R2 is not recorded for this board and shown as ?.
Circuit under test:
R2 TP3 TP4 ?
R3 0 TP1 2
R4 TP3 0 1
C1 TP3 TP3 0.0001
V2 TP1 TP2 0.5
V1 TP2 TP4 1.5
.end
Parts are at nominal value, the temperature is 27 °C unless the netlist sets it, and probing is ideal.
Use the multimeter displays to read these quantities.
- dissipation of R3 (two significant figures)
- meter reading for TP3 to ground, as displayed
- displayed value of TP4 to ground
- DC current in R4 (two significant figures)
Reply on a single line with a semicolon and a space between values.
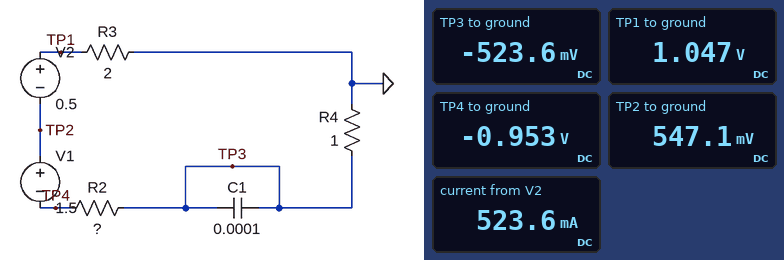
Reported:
550 mW; -523.6 mV; -0.953 V; 520 mA
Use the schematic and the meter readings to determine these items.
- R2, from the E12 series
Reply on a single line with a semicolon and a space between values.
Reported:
0.82 Ω
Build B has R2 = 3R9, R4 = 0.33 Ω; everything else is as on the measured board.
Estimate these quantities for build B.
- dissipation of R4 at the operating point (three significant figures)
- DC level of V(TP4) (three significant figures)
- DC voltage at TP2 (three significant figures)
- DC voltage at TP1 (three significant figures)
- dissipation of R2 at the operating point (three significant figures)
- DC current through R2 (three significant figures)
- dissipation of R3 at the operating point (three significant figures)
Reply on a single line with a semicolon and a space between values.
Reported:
34.0 mW; -1.36 V; 142 mV; 642 mV; 402 mW; 321 mA; 206 mW
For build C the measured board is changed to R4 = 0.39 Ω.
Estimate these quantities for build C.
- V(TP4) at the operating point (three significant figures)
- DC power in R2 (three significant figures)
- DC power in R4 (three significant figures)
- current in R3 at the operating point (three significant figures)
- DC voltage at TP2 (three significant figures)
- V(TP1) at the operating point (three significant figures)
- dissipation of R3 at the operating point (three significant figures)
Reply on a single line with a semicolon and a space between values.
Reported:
-754 mV; 318 mW; 151 mW; 623 mA; 746 mV; 1.25 V; 776 mW
